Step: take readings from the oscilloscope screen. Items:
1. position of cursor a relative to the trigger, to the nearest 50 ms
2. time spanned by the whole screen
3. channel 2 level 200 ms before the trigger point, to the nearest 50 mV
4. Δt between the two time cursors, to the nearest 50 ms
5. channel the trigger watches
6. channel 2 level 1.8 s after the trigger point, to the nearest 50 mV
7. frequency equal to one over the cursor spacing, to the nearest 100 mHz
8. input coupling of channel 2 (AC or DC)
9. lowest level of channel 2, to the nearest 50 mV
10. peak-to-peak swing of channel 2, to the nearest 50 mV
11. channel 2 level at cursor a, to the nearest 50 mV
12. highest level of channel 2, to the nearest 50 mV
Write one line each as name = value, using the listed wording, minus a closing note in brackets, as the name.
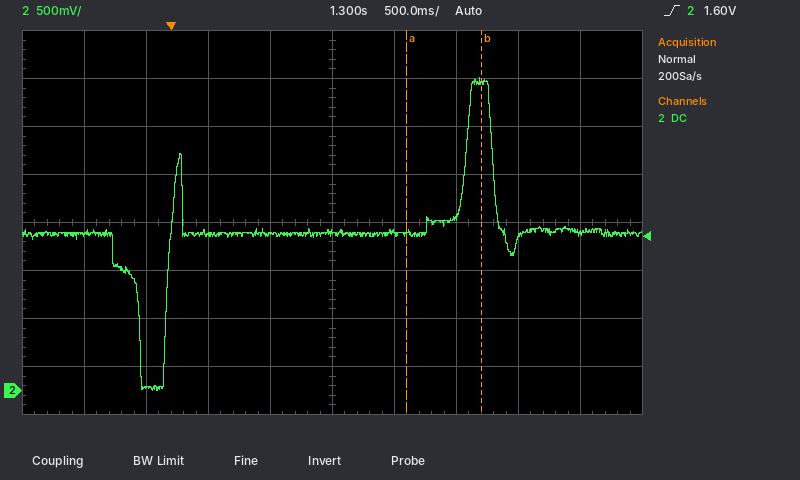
position of cursor a relative to the trigger, to the nearest 50 ms = +1.90 s
time spanned by the whole screen = 5 s
channel 2 level 200 ms before the trigger point, to the nearest 50 mV = 50 mV
Δt between the two time cursors, to the nearest 50 ms = 600 ms
channel the trigger watches = channel 2
channel 2 level 1.8 s after the trigger point, to the nearest 50 mV = 1.65 V
frequency equal to one over the cursor spacing, to the nearest 100 mHz = 1.7 Hz
input coupling of channel 2 = DC
lowest level of channel 2, to the nearest 50 mV = 0 mV
peak-to-peak swing of channel 2, to the nearest 50 mV = 3.25 V
channel 2 level at cursor a, to the nearest 50 mV = 1.65 V
highest level of channel 2, to the nearest 50 mV = 3.25 V
